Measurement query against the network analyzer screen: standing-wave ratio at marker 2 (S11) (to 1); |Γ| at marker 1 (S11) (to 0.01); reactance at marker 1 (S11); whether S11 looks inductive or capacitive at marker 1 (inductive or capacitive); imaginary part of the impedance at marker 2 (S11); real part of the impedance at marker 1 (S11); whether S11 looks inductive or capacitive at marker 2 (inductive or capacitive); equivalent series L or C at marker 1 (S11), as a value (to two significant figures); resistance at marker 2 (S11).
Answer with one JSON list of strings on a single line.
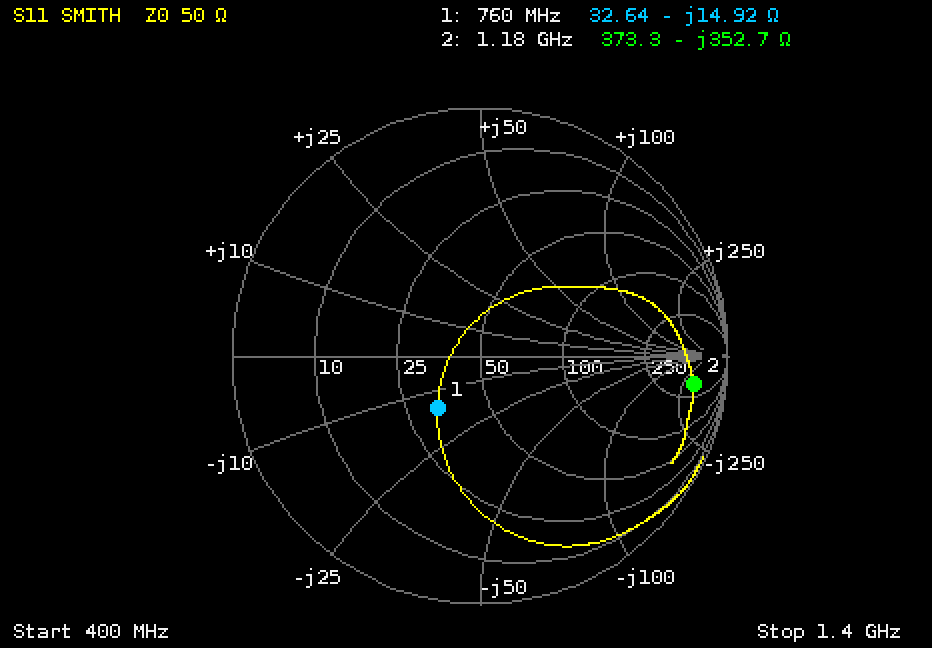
["14", "0.27", "-14.92 Ω", "capacitive", "-352.7 Ω", "32.64 Ω", "capacitive", "14 pF", "373.3 Ω"]
